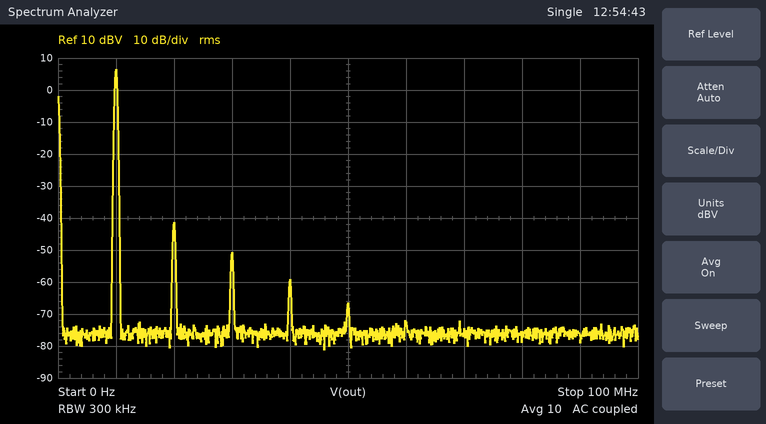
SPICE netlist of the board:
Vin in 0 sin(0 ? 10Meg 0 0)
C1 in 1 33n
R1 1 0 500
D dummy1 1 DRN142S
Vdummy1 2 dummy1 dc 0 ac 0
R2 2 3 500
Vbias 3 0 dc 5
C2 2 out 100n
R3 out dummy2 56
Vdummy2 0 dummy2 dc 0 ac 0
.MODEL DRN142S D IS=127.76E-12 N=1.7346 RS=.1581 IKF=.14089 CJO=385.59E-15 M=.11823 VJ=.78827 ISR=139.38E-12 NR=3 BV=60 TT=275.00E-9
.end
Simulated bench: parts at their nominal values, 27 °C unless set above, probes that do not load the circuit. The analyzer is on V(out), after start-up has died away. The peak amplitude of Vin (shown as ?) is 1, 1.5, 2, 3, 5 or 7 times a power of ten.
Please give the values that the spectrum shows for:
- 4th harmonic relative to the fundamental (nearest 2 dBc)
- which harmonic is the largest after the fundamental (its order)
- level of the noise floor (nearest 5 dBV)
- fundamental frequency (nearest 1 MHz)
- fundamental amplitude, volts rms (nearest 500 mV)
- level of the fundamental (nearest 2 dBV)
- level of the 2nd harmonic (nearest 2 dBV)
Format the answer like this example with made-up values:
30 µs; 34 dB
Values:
-66 dBc; 2; -75 dBV; 10 MHz; 2.0 V; 6 dBV; -42 dBV
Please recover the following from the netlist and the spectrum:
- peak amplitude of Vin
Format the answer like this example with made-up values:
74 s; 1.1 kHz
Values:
3 V
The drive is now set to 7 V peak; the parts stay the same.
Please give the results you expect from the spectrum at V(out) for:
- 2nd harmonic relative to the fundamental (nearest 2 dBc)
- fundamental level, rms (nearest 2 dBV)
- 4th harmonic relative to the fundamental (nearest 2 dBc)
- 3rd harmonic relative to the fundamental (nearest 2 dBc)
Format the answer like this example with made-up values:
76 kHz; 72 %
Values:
-12 dBc; 12 dBV; -18 dBc; -14 dBc
